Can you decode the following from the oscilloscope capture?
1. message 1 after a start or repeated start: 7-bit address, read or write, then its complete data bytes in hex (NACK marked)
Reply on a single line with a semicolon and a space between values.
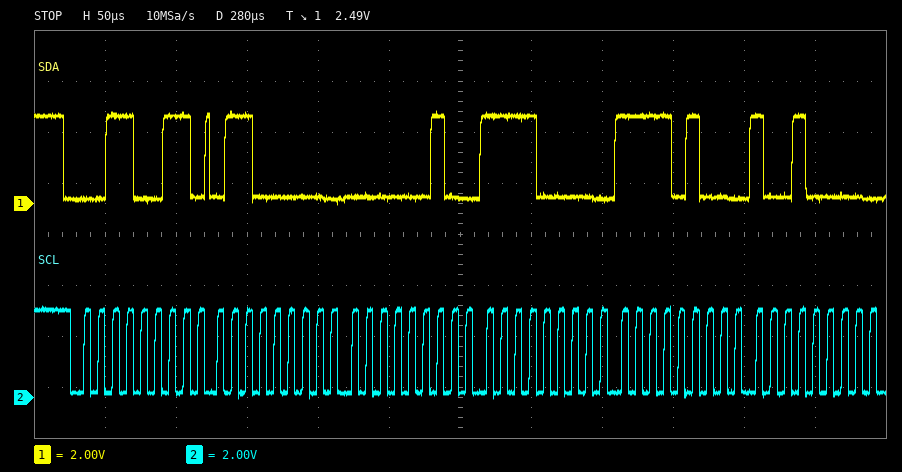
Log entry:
0x19 read: 60 02 F0 F4 90
